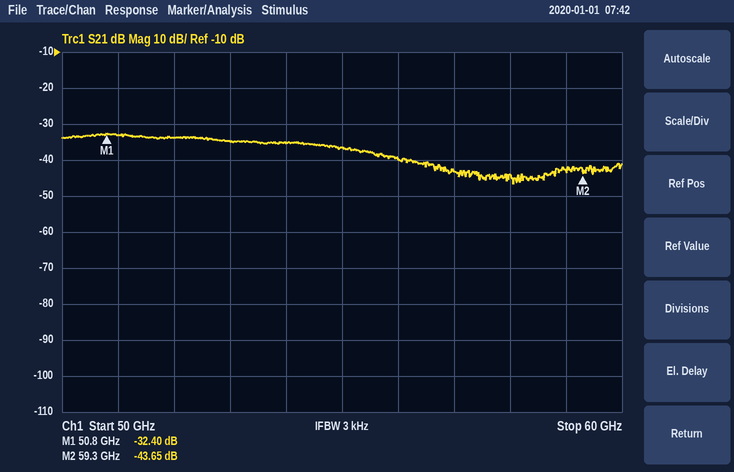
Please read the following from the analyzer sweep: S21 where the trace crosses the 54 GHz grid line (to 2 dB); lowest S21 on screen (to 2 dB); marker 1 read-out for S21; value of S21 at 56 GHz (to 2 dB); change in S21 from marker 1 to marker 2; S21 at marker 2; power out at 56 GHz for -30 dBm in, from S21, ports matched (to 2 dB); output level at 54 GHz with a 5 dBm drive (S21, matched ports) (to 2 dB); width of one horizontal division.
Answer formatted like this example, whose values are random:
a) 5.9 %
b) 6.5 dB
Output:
a) -36 dB
b) -46 dB
c) -32.40 dB
d) -40 dB
e) -11.25 dB
f) -43.65 dB
g) -70 dBm
h) -30 dBm
i) 1 GHz
